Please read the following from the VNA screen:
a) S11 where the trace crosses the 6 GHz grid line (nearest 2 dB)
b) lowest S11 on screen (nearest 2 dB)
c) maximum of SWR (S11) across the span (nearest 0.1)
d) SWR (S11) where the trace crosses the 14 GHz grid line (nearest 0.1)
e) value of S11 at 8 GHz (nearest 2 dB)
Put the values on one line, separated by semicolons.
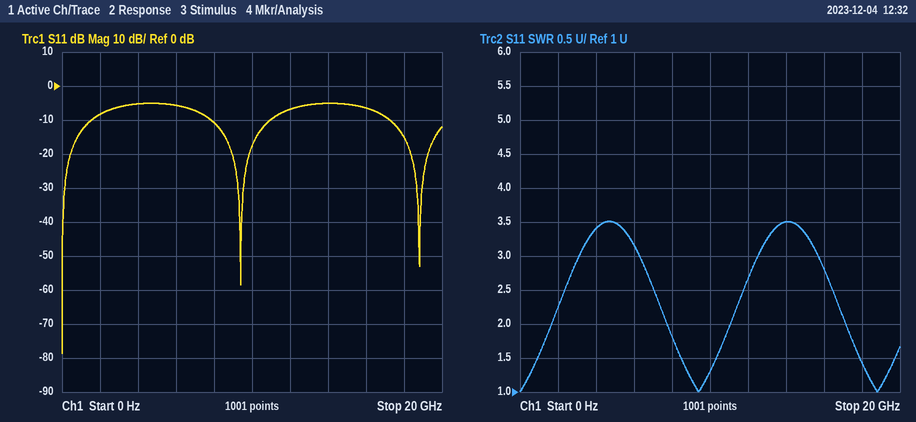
-6 dB; -78 dB; 3.5; 3.5; -10 dB
